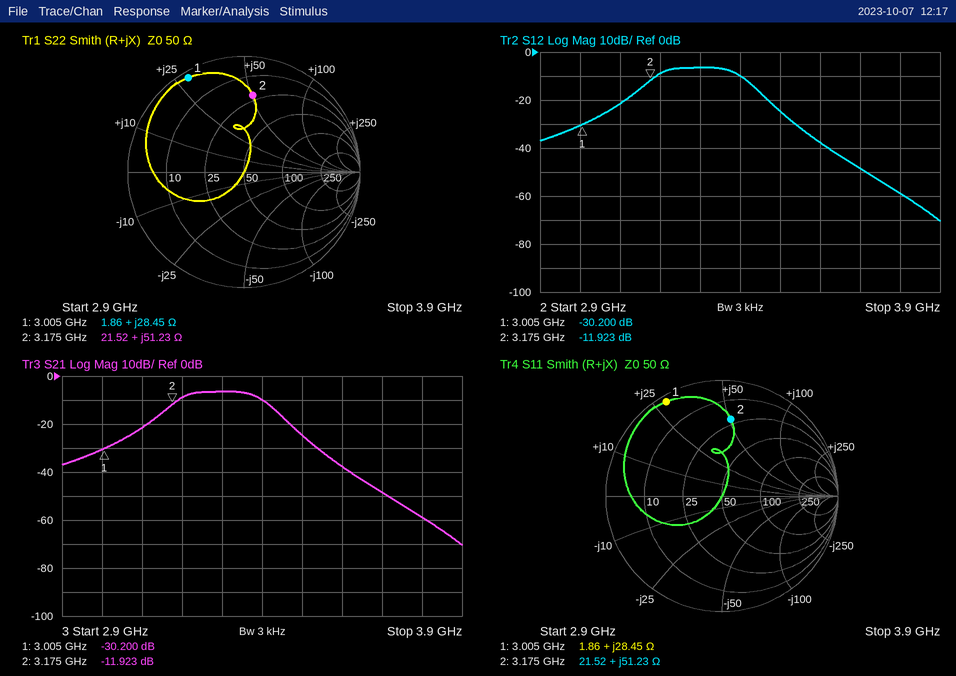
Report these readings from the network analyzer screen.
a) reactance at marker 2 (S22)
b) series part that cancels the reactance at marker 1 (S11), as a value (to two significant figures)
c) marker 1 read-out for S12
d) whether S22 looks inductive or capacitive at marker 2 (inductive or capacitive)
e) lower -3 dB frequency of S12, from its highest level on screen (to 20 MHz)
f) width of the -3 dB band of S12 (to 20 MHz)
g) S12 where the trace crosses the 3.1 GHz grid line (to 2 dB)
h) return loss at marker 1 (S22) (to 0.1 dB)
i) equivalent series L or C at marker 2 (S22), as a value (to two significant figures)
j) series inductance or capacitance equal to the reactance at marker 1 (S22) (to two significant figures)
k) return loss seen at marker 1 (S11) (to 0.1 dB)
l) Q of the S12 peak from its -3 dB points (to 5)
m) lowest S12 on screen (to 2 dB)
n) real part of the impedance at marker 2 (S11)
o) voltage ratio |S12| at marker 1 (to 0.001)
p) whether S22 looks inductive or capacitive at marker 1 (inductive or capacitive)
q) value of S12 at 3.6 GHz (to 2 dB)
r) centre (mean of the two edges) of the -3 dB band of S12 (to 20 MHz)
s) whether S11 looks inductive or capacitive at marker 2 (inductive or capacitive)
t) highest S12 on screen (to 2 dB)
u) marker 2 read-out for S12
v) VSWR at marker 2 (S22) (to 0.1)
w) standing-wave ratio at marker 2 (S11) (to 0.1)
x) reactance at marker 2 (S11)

+51.23 Ω
1.9 pF
-30.200 dB
inductive
3.20 GHz
200 MHz
-22 dB
0.5 dB
2.6 nH
1.5 nH
0.5 dB
15
-70 dB
21.52 Ω
0.031
inductive
-38 dB
3.30 GHz
inductive
-6 dB
-11.923 dB
5.0
5.0
+51.23 Ω
